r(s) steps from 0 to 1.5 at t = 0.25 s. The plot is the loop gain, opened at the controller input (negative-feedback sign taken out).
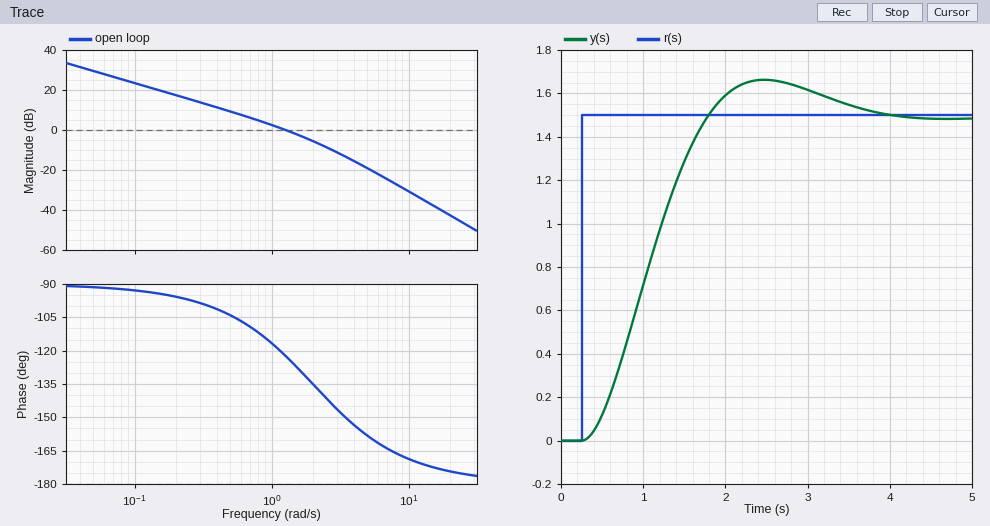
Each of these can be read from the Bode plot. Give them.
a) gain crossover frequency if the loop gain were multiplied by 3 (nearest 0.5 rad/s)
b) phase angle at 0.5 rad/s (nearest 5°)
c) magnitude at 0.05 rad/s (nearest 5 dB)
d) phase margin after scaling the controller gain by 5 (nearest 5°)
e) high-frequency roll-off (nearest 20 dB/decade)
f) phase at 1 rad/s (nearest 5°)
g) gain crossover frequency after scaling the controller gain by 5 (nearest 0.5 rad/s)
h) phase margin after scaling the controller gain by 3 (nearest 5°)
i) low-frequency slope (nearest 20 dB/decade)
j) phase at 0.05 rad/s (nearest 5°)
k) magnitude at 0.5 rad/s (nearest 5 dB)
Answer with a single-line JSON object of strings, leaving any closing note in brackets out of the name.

{"gain crossover frequency if the loop gain were multiplied by 3": "2.5 rad/s", "phase angle at 0.5 rad/s": "-105°", "magnitude at 0.05 rad/s": "30 dB", "phase margin after scaling the controller gain by 5": "30°", "high-frequency roll-off": "-40 dB/decade", "phase at 1 rad/s": "-115°", "gain crossover frequency after scaling the controller gain by 5": "3.5 rad/s", "phase margin after scaling the controller gain by 3": "35°", "low-frequency slope": "-20 dB/decade", "phase at 0.05 rad/s": "-90°", "magnitude at 0.5 rad/s": "10 dB"}
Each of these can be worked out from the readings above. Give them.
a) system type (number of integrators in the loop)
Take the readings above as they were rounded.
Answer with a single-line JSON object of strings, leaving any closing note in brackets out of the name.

{"system type": "1"}
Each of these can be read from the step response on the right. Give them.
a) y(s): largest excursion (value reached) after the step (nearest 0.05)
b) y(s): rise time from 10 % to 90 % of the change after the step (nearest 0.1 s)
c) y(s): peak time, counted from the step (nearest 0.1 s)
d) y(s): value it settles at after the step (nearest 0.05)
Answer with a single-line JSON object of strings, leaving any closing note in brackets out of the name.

{"y(s): largest excursion (value reached) after the step": "1.65", "y(s): rise time from 10 % to 90 % of the change after the step": "1.0 s", "y(s): peak time, counted from the step": "2.2 s", "y(s): value it settles at after the step": "1.50"}
